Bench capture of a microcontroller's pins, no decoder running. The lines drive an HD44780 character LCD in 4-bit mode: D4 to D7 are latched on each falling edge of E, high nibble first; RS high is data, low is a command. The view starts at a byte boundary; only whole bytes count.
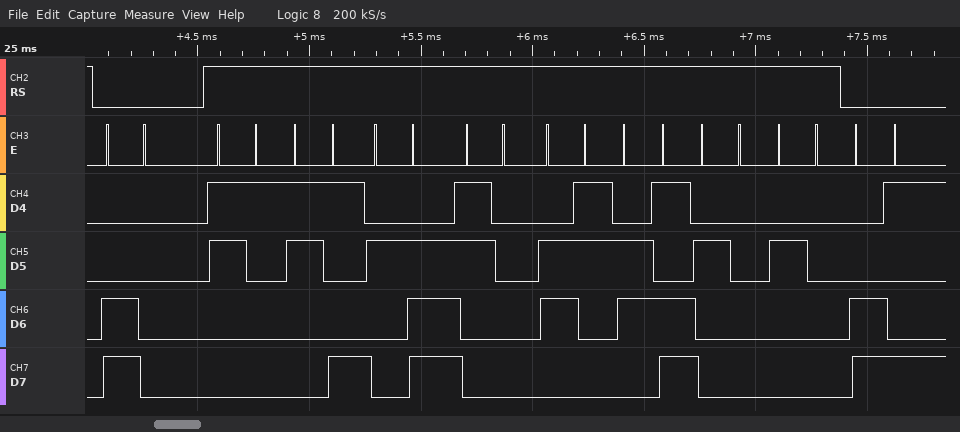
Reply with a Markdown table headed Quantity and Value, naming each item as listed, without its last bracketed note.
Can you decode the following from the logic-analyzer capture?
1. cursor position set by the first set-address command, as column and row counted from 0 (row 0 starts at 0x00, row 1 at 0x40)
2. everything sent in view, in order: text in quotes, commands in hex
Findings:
| Quantity | Value |
|---|---|
| cursor position set by the first set-address command, as column and row counted from 0 | column 0, row 1 |
| everything sent in view, in order: text in quotes, commands in hex | 0xC0 "19.0cm  " 0xC9 |
